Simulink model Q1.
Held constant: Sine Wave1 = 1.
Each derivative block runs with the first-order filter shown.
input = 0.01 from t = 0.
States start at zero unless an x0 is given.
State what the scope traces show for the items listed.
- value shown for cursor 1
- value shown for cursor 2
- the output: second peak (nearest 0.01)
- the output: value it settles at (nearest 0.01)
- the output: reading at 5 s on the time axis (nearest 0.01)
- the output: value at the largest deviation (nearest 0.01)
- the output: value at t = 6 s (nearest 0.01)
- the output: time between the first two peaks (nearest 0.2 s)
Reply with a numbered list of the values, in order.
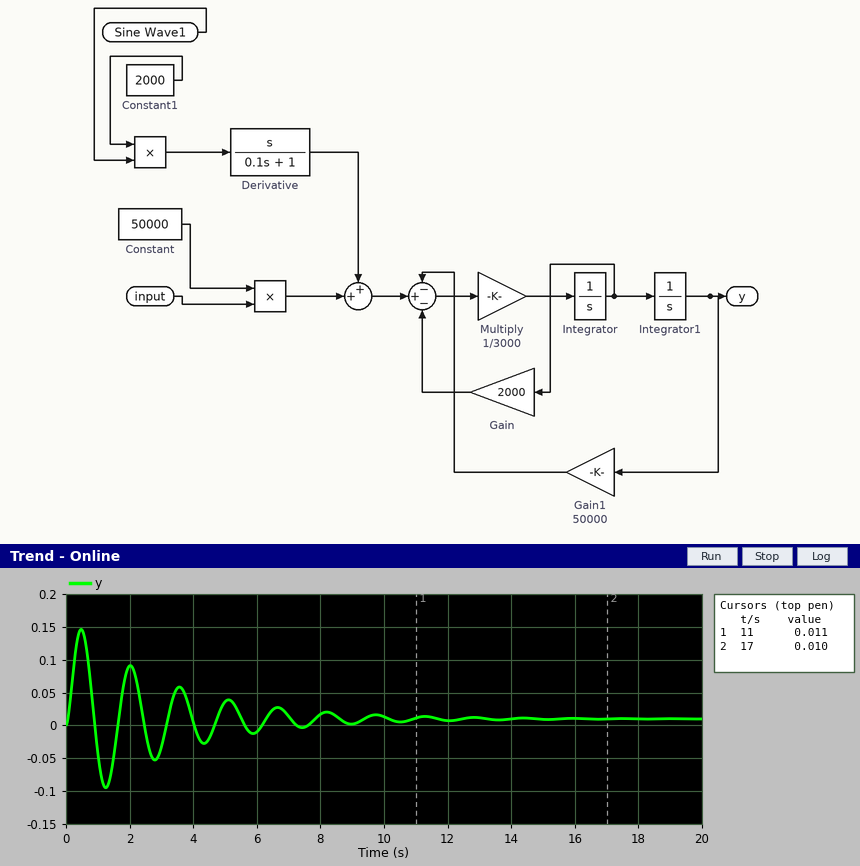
1. 0.011
2. 0.010
3. 0.09
4. 0.01
5. 0.04
6. 0.15
7. -0.01
8. 1.6 s
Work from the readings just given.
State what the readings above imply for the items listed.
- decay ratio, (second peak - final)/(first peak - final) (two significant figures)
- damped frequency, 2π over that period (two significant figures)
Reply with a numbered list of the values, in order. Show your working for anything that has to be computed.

1. (0.09 - 0.01) / (0.15 - 0.01) = 0.57
2. 2π / 1.6 = 3.9 rad/s
